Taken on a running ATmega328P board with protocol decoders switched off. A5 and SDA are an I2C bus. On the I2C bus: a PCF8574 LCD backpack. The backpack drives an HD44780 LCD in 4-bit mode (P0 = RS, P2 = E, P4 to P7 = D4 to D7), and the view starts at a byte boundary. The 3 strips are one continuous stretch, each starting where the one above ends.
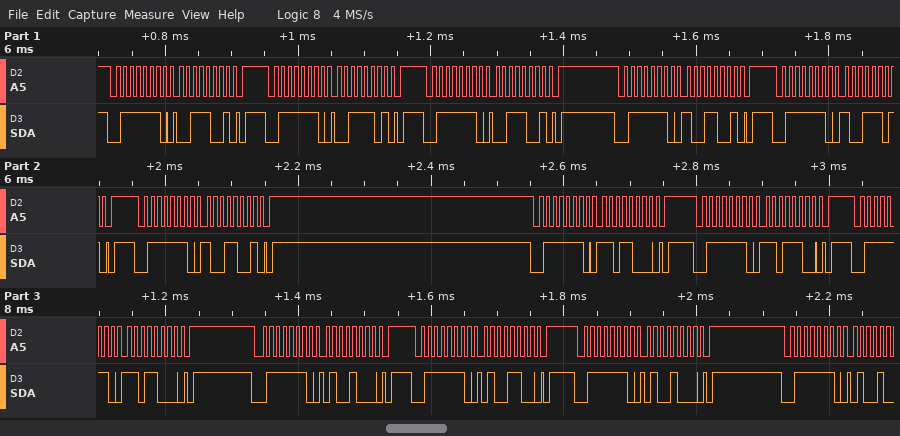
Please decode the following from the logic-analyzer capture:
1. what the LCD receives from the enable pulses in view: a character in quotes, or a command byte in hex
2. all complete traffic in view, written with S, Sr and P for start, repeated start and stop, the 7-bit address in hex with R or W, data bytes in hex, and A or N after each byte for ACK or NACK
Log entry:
'9' 0xD4
S 3FW A 39 A P S 3FW A 3D A P S 3FW A 39 A P S 3FW A 99 A P S 3FW A 9D A P S 3FW A 99 A P S 3FW A D8 A P S 3FW A DC A P S 3FW A D8 A P S 3FW A 48 A P S 3FW A 4C A P S 3FW A 48 A P S 3FW A
